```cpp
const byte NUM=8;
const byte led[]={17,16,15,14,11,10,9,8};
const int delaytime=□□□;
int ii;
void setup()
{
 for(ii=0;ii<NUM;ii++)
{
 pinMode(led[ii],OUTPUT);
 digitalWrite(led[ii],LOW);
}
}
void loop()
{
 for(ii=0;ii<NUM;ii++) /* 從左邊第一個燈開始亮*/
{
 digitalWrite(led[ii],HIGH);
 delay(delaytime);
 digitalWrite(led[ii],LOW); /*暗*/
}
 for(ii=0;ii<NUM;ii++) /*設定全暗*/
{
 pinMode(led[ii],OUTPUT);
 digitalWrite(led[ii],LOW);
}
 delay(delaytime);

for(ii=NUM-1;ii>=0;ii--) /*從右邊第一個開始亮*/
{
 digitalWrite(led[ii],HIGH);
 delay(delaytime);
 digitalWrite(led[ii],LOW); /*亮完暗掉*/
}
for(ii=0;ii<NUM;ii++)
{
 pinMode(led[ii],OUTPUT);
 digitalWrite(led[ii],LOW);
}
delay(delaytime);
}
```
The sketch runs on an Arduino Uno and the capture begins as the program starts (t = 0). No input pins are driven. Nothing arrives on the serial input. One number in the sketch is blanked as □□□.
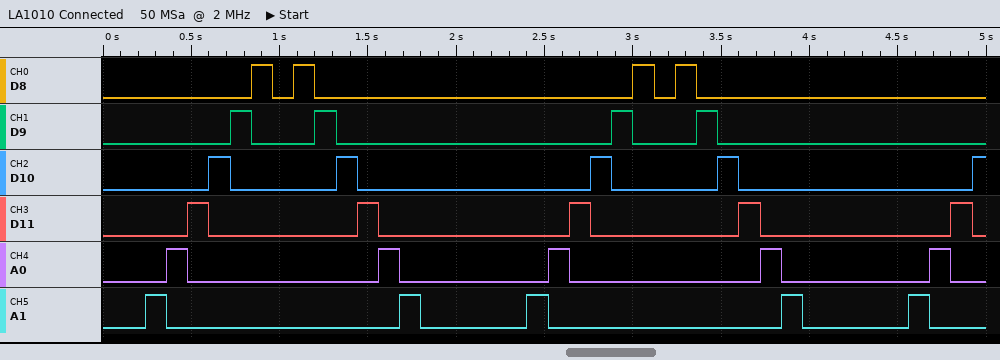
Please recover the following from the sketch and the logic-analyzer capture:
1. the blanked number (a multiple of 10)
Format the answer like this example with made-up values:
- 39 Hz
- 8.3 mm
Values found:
- 120
